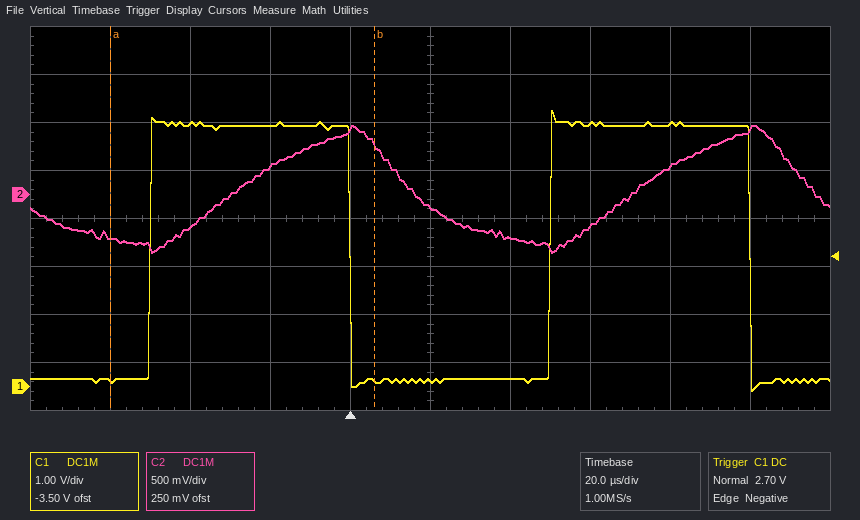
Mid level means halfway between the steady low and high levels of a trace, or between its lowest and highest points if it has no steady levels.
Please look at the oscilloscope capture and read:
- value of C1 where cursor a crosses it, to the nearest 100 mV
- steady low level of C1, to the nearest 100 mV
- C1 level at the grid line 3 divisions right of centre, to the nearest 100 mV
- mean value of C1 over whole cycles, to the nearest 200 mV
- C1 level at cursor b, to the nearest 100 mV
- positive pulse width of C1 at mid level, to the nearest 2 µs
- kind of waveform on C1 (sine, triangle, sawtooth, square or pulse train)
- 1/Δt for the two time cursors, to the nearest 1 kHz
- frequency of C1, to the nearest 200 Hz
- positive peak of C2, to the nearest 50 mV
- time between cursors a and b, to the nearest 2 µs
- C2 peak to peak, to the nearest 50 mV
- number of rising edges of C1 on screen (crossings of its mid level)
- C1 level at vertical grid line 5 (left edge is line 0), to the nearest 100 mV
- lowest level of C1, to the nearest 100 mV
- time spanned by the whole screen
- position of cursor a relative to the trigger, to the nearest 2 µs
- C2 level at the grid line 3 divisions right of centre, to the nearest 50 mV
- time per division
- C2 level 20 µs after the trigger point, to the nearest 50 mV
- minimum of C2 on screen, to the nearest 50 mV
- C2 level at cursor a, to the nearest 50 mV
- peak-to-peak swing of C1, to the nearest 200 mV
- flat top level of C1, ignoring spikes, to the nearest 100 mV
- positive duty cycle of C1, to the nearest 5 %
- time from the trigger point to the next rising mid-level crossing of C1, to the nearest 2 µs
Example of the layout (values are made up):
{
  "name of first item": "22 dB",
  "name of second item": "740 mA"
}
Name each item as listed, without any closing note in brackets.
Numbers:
{
  "value of C1 where cursor a crosses it, to the nearest 100 mV": "100 mV",
  "steady low level of C1, to the nearest 100 mV": "200 mV",
  "C1 level at the grid line 3 divisions right of centre, to the nearest 100 mV": "5.5 V",
  "mean value of C1 over whole cycles, to the nearest 200 mV": "2.8 V",
  "C1 level at cursor b, to the nearest 100 mV": "100 mV",
  "positive pulse width of C1 at mid level, to the nearest 2 µs": "50 µs",
  "kind of waveform on C1": "square",
  "1/Δt for the two time cursors, to the nearest 1 kHz": "15 kHz",
  "frequency of C1, to the nearest 200 Hz": "10.0 kHz",
  "positive peak of C2, to the nearest 50 mV": "700 mV",
  "time between cursors a and b, to the nearest 2 µs": "66 µs",
  "C2 peak to peak, to the nearest 50 mV": "1.30 V",
  "number of rising edges of C1 on screen": "2",
  "C1 level at vertical grid line 5 (left edge is line 0), to the nearest 100 mV": "100 mV",
  "lowest level of C1, to the nearest 100 mV": "-100 mV",
  "time spanned by the whole screen": "200 µs",
  "position of cursor a relative to the trigger, to the nearest 2 µs": "-60 µs",
  "C2 level at the grid line 3 divisions right of centre, to the nearest 50 mV": "300 mV",
  "time per division": "20 µs",
  "C2 level 20 µs after the trigger point, to the nearest 50 mV": "-150 mV",
  "minimum of C2 on screen, to the nearest 50 mV": "-600 mV",
  "C2 level at cursor a, to the nearest 50 mV": "-450 mV",
  "peak-to-peak swing of C1, to the nearest 200 mV": "5.8 V",
  "flat top level of C1, ignoring spikes, to the nearest 100 mV": "5.4 V",
  "positive duty cycle of C1, to the nearest 5 %": "50 %",
  "time from the trigger point to the next rising mid-level crossing of C1, to the nearest 2 µs": "50 µs"
}
